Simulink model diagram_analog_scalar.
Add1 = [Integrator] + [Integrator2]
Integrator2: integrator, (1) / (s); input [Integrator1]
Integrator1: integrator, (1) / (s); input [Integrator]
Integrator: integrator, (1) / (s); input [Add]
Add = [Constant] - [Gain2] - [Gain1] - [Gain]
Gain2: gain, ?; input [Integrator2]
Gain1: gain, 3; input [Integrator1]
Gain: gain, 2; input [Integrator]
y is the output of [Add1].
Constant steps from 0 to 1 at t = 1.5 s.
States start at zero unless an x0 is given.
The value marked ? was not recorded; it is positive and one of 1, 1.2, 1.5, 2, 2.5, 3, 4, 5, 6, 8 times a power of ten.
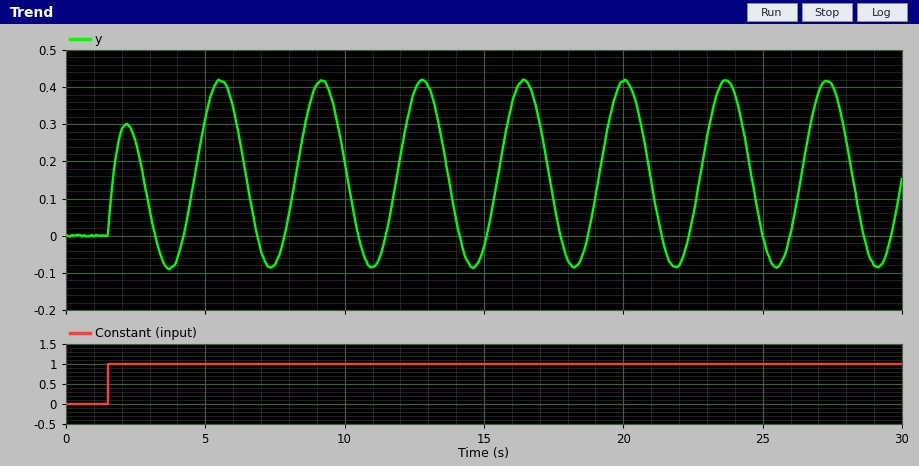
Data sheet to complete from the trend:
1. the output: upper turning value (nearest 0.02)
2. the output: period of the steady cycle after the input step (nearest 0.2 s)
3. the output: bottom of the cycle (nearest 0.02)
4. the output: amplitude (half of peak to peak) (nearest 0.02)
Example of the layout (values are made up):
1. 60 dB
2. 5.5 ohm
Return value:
1. 0.42
2. 3.6 s
3. -0.08
4. 0.26
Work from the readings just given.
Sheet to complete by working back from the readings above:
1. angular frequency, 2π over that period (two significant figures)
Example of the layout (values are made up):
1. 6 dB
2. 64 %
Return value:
1. 1.7 rad/s
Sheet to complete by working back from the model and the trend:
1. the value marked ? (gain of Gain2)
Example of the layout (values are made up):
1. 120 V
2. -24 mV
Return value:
1. 6
